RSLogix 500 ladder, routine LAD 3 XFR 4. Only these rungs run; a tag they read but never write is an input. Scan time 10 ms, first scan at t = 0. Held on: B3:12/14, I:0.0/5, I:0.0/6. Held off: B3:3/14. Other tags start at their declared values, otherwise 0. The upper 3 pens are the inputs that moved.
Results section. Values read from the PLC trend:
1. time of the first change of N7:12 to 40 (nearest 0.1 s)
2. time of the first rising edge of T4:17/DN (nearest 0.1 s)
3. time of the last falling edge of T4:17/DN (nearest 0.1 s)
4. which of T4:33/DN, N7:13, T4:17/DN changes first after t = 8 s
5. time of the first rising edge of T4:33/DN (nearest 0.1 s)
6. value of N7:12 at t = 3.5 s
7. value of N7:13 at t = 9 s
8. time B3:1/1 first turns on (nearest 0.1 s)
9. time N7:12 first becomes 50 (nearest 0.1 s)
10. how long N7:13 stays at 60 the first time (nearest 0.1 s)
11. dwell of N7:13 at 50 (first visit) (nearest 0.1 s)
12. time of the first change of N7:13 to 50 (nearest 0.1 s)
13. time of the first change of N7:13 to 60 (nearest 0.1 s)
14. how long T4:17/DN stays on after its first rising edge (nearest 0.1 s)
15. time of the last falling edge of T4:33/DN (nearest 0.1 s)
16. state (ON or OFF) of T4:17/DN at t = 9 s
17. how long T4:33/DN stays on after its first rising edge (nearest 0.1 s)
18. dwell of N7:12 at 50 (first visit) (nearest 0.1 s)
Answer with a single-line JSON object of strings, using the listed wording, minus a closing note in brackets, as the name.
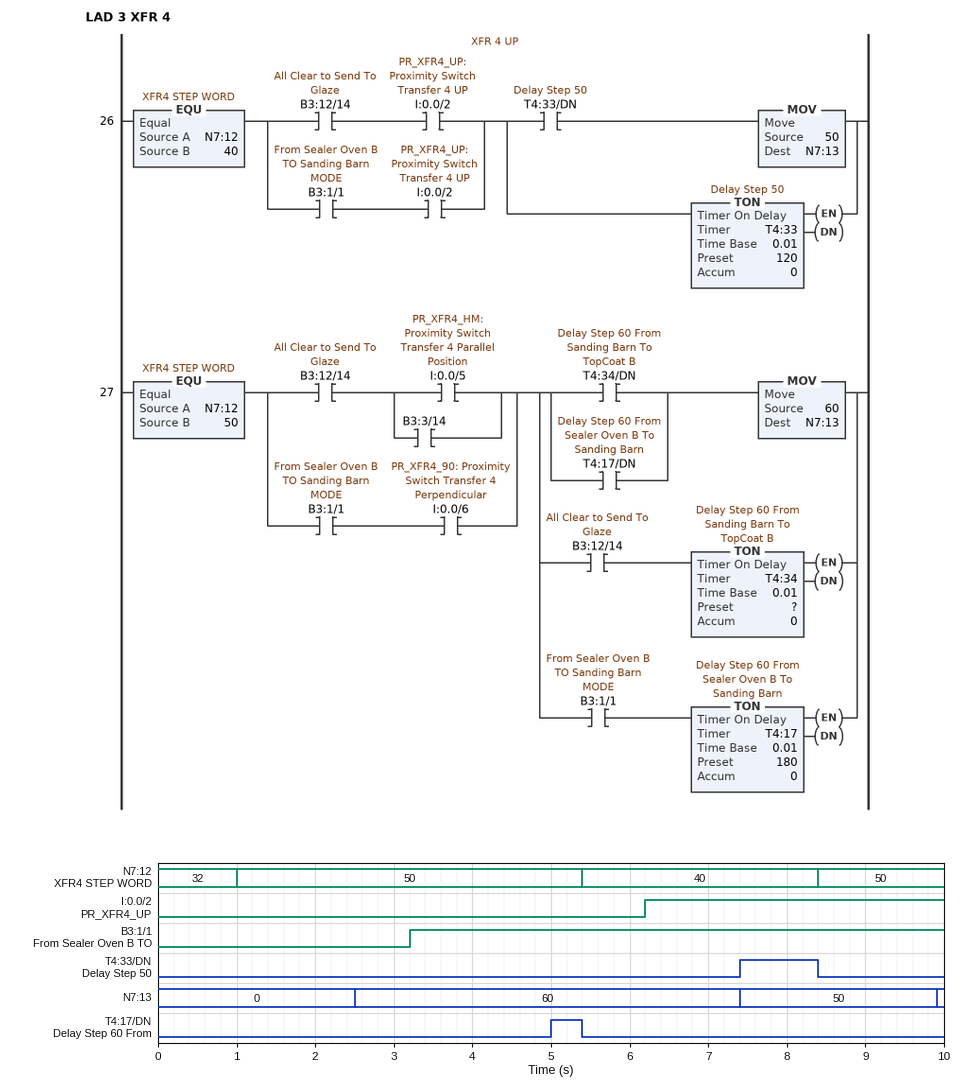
{"time of the first change of N7:12 to 40": "5.4 s", "time of the first rising edge of T4:17/DN": "5.0 s", "time of the last falling edge of T4:17/DN": "5.4 s", "which of T4:33/DN, N7:13, T4:17/DN changes first after t = 8 s": "T4:33/DN", "time of the first rising edge of T4:33/DN": "7.4 s", "value of N7:12 at t = 3.5 s": "50", "value of N7:13 at t = 9 s": "50", "time B3:1/1 first turns on": "3.2 s", "time N7:12 first becomes 50": "1.0 s", "how long N7:13 stays at 60 the first time": "4.9 s", "dwell of N7:13 at 50 (first visit)": "2.5 s", "time of the first change of N7:13 to 50": "7.4 s", "time of the first change of N7:13 to 60": "2.5 s", "how long T4:17/DN stays on after its first rising edge": "0.4 s", "time of the last falling edge of T4:33/DN": "8.4 s", "state (ON or OFF) of T4:17/DN at t = 9 s": "OFF", "how long T4:33/DN stays on after its first rising edge": "1.0 s", "dwell of N7:12 at 50 (first visit)": "4.4 s"}
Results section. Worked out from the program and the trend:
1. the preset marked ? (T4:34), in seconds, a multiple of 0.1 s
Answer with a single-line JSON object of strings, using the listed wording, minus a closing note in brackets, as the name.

{"the preset marked ? (T4:34), in seconds, a multiple of 0.1 s": "1.5 s"}
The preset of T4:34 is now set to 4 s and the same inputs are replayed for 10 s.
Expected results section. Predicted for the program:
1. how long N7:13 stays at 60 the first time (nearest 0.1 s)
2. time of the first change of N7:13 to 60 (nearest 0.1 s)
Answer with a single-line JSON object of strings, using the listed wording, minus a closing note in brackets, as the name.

{"how long N7:13 stays at 60 the first time": "2.4 s", "time of the first change of N7:13 to 60": "5.0 s"}
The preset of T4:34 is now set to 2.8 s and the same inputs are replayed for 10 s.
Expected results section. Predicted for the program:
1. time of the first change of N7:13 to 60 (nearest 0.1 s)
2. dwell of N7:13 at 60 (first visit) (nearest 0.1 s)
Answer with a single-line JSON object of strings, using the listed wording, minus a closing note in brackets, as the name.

{"time of the first change of N7:13 to 60": "3.8 s", "dwell of N7:13 at 60 (first visit)": "3.6 s"}
